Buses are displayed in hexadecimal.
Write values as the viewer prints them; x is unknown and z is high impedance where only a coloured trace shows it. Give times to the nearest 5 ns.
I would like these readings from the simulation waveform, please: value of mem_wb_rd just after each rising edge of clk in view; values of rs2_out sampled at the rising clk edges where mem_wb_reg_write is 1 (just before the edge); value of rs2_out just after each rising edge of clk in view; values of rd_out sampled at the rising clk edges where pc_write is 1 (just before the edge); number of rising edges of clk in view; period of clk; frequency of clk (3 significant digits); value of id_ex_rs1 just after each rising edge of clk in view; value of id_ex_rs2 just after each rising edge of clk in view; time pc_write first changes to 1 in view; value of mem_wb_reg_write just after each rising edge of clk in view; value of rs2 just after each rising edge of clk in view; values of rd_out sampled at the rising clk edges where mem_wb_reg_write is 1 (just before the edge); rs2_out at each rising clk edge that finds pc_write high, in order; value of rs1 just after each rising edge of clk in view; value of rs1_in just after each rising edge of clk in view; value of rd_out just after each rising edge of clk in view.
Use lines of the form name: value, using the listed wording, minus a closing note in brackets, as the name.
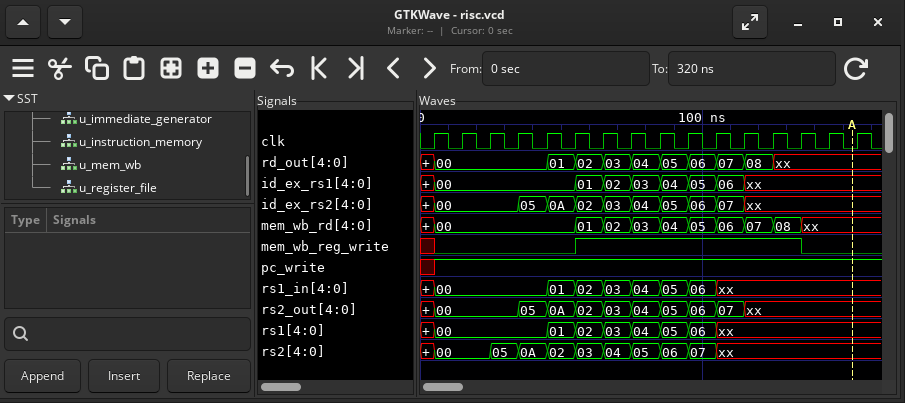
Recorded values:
value of mem_wb_rd just after each rising edge of clk in view: 00, 00, 00, 00, 00, 01, 02, 03, 04, 05, 06, 07, 08, xx, xx, xx
values of rs2_out sampled at the rising clk edges where mem_wb_reg_write is 1: 02, 03, 04, 05, 06, 07, xx, xx
value of rs2_out just after each rising edge of clk in view: 00, 00, 00, 05, 0A, 02, 03, 04, 05, 06, 07, xx, xx, xx, xx, xx
values of rd_out sampled at the rising clk edges where pc_write is 1: 00, 00, 00, 00, 01, 02, 03, 04, 05, 06, 07, 08, xx, xx, xx
number of rising edges of clk in view: 16
period of clk: 10 ns
frequency of clk: 100 MHz
value of id_ex_rs1 just after each rising edge of clk in view: 00, 00, 00, 00, 00, 01, 02, 03, 04, 05, 06, xx, xx, xx, xx, xx
value of id_ex_rs2 just after each rising edge of clk in view: 00, 00, 00, 05, 0A, 02, 03, 04, 05, 06, 07, xx, xx, xx, xx, xx
time pc_write first changes to 1 in view: 5 ns
value of mem_wb_reg_write just after each rising edge of clk in view: 0 0 0 0 0 1 1 1 1 1 1 1 1 0 0 0
value of rs2 just after each rising edge of clk in view: 00, 00, 05, 0A, 02, 03, 04, 05, 06, 07, xx, xx, xx, xx, xx, xx
values of rd_out sampled at the rising clk edges where mem_wb_reg_write is 1: 02, 03, 04, 05, 06, 07, 08, xx
rs2_out at each rising clk edge that finds pc_write high, in order: 00, 00, 00, 05, 0A, 02, 03, 04, 05, 06, 07, xx, xx, xx, xx
value of rs1 just after each rising edge of clk in view: 00, 00, 00, 00, 01, 02, 03, 04, 05, 06, xx, xx, xx, xx, xx, xx
value of rs1_in just after each rising edge of clk in view: 00, 00, 00, 00, 01, 02, 03, 04, 05, 06, xx, xx, xx, xx, xx, xx
value of rd_out just after each rising edge of clk in view: 00, 00, 00, 00, 01, 02, 03, 04, 05, 06, 07, 08, xx, xx, xx, xx
